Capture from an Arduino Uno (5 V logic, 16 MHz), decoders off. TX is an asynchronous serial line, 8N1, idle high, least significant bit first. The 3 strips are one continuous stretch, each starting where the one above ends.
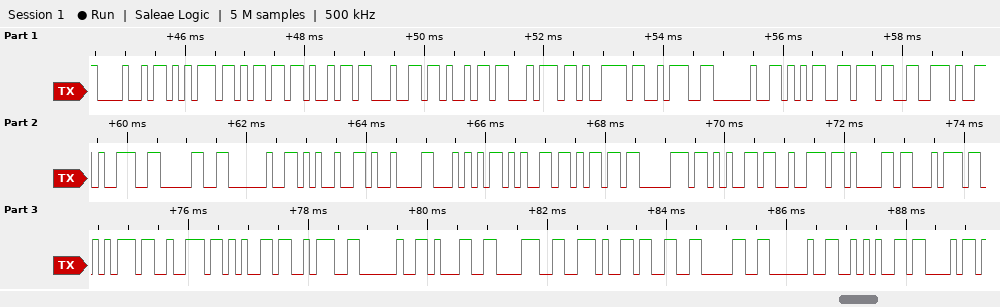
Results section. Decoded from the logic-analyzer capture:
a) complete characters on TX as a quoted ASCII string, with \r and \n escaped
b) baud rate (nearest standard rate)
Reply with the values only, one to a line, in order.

"Humidity: 57.90 %\tTemperature: 18.30 *C"
9600 baud
